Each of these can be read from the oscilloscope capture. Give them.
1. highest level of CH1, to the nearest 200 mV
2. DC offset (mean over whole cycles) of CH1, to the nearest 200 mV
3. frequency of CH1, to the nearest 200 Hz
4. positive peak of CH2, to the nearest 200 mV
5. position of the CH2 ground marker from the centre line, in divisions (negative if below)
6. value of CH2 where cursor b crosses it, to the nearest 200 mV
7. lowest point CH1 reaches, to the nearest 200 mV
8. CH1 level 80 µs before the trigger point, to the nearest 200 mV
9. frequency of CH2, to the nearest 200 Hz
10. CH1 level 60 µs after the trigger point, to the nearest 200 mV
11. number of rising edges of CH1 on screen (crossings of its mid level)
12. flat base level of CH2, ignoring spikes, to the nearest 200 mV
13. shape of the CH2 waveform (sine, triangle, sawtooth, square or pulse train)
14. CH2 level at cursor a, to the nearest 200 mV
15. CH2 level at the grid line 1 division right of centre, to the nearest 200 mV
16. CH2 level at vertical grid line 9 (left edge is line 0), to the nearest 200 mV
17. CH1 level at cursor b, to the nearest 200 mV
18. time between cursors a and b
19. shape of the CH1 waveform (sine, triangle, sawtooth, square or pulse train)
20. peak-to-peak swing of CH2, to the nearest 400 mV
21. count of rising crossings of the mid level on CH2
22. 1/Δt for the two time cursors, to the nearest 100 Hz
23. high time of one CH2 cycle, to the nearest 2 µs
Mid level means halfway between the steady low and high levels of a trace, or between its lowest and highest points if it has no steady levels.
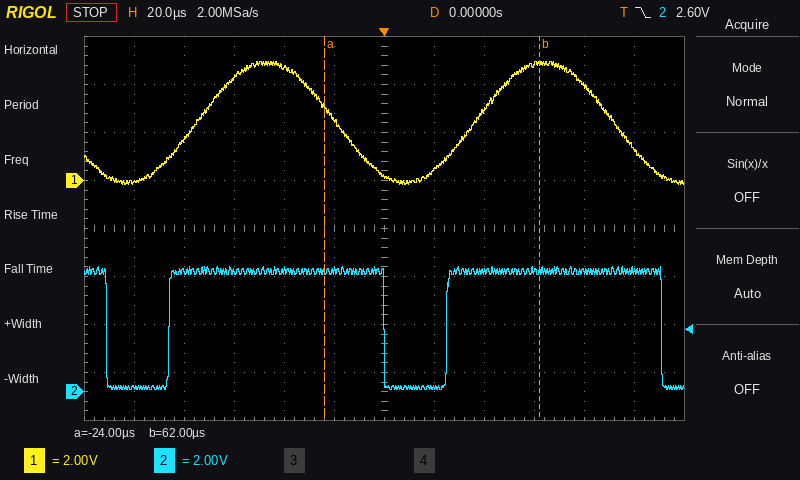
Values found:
5.0 V
2.4 V
9.0 kHz
5.2 V
-3.4 div
5.0 V
-200 mV
1.8 V
9.0 kHz
4.8 V
2
200 mV
pulse train
5.0 V
200 mV
5.0 V
4.8 V
86 µs
sine
5.2 V
2
11.6 kHz
86 µs
